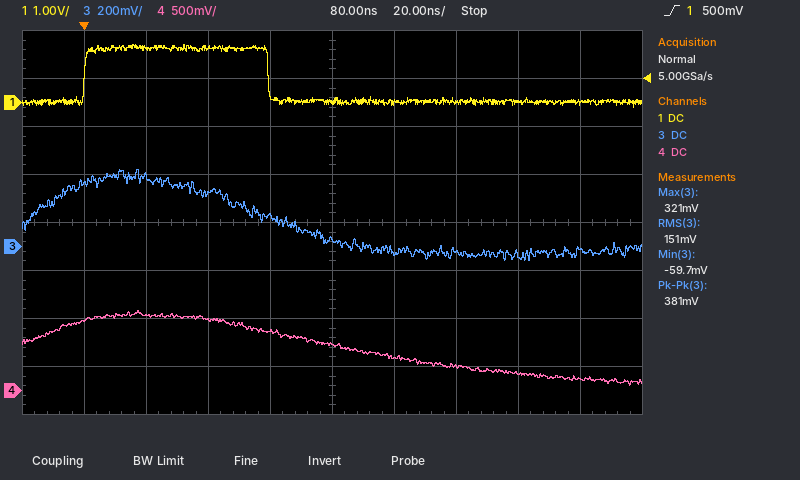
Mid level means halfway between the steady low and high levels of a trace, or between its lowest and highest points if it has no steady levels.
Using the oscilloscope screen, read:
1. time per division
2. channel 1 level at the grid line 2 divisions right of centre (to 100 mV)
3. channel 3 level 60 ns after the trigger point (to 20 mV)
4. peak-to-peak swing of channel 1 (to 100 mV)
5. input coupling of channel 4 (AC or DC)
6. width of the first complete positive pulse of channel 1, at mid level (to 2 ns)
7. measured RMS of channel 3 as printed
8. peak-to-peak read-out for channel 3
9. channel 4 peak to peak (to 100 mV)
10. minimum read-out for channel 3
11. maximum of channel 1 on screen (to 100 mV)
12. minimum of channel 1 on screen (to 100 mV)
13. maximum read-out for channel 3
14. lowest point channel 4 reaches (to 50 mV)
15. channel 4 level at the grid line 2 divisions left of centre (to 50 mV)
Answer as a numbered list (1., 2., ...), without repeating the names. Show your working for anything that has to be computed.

1. 20 ns
2. 0.0 V
3. 120 mV
4. 1.2 V − (-100 mV) = 1.3 V
5. DC
6. 60 ns
7. 151 mV
8. 381 mV
9. 800 mV
10. -59.7 mV
11. 1.2 V
12. -100 mV
13. 321 mV
14. 50 mV
15. 750 mV
